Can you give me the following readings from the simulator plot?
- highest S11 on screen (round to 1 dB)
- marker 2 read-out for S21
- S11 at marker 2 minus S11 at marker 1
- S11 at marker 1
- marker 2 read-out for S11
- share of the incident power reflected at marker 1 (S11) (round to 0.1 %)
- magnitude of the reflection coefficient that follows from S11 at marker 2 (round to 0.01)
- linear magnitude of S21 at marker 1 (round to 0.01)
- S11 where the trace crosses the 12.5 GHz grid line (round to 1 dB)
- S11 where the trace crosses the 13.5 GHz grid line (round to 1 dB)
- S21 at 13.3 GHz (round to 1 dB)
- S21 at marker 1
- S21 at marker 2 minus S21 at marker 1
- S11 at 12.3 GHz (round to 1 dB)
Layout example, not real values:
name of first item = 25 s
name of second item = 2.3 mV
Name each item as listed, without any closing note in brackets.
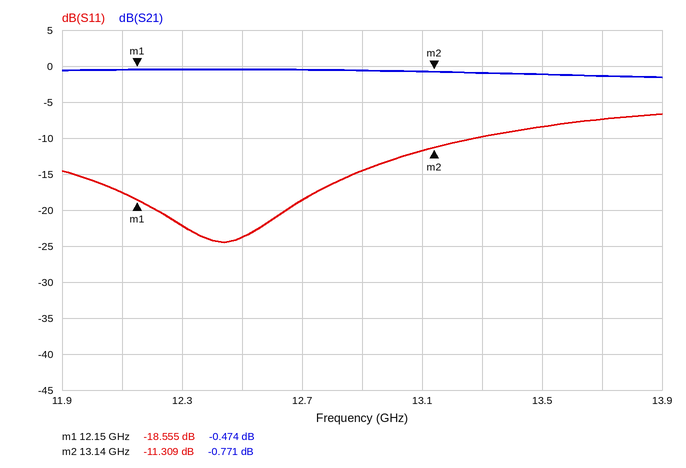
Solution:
highest S11 on screen = -7 dB
marker 2 read-out for S21 = -0.771 dB
S11 at marker 2 minus S11 at marker 1 = 7.246 dB
S11 at marker 1 = -18.555 dB
marker 2 read-out for S11 = -11.309 dB
share of the incident power reflected at marker 1 (S11) = 1.4 %
magnitude of the reflection coefficient that follows from S11 at marker 2 = 0.27
linear magnitude of S21 at marker 1 = 0.95
S11 where the trace crosses the 12.5 GHz grid line = -24 dB
S11 where the trace crosses the 13.5 GHz grid line = -8 dB
S21 at 13.3 GHz = -1 dB
S21 at marker 1 = -0.474 dB
S21 at marker 2 minus S21 at marker 1 = -0.297 dB
S11 at 12.3 GHz = -22 dB
